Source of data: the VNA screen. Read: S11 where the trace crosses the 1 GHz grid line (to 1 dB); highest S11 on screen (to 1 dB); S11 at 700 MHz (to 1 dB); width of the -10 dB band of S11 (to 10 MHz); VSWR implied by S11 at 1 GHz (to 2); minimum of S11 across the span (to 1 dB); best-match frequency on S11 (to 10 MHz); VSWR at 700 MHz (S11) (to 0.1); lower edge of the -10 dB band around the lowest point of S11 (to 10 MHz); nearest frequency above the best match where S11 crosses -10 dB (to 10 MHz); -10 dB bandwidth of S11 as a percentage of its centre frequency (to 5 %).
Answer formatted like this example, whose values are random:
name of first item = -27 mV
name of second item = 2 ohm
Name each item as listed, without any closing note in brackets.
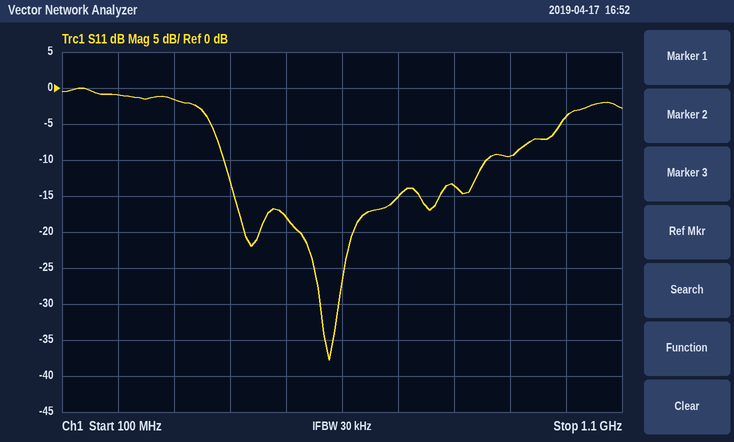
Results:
S11 where the trace crosses the 1 GHz grid line = -4 dB
highest S11 on screen = 0 dB
S11 at 700 MHz = -15 dB
width of the -10 dB band of S11 = 470 MHz
VSWR implied by S11 at 1 GHz = 4
minimum of S11 across the span = -38 dB
best-match frequency on S11 = 580 MHz
VSWR at 700 MHz (S11) = 1.4
lower edge of the -10 dB band around the lowest point of S11 = 390 MHz
nearest frequency above the best match where S11 crosses -10 dB = 860 MHz
-10 dB bandwidth of S11 as a percentage of its centre frequency = 75 %
